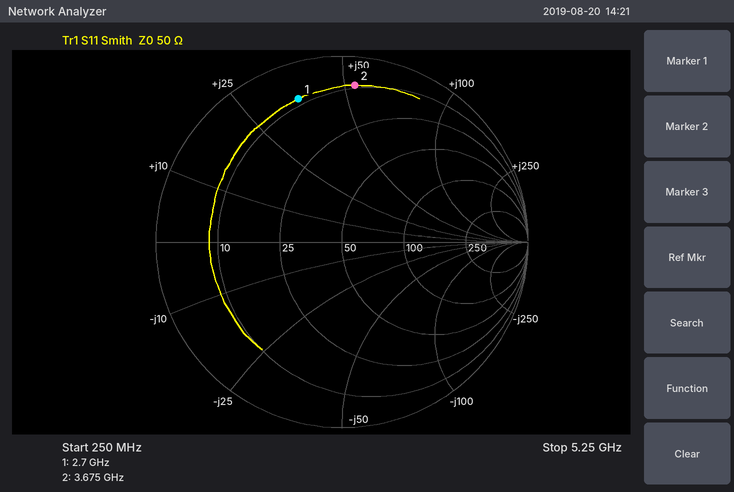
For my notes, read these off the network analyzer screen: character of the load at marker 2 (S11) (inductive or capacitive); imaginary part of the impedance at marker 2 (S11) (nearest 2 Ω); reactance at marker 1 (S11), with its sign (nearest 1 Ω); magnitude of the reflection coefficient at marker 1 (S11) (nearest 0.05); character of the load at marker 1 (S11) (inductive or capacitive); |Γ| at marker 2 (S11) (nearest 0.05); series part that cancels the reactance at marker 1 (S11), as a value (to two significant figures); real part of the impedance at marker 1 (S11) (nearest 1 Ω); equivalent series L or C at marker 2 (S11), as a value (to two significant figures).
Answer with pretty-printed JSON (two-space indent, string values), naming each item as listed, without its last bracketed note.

{
  "character of the load at marker 2 (S11)": "inductive",
  "imaginary part of the impedance at marker 2 (S11)": "+54 Ω",
  "reactance at marker 1 (S11), with its sign": "+36 Ω",
  "magnitude of the reflection coefficient at marker 1 (S11)": "0.80",
  "character of the load at marker 1 (S11)": "inductive",
  "|Γ| at marker 2 (S11)": "0.85",
  "series part that cancels the reactance at marker 1 (S11), as a value": "1.6 pF",
  "real part of the impedance at marker 1 (S11)": "8 Ω",
  "equivalent series L or C at marker 2 (S11), as a value": "2.3 nH"
}
